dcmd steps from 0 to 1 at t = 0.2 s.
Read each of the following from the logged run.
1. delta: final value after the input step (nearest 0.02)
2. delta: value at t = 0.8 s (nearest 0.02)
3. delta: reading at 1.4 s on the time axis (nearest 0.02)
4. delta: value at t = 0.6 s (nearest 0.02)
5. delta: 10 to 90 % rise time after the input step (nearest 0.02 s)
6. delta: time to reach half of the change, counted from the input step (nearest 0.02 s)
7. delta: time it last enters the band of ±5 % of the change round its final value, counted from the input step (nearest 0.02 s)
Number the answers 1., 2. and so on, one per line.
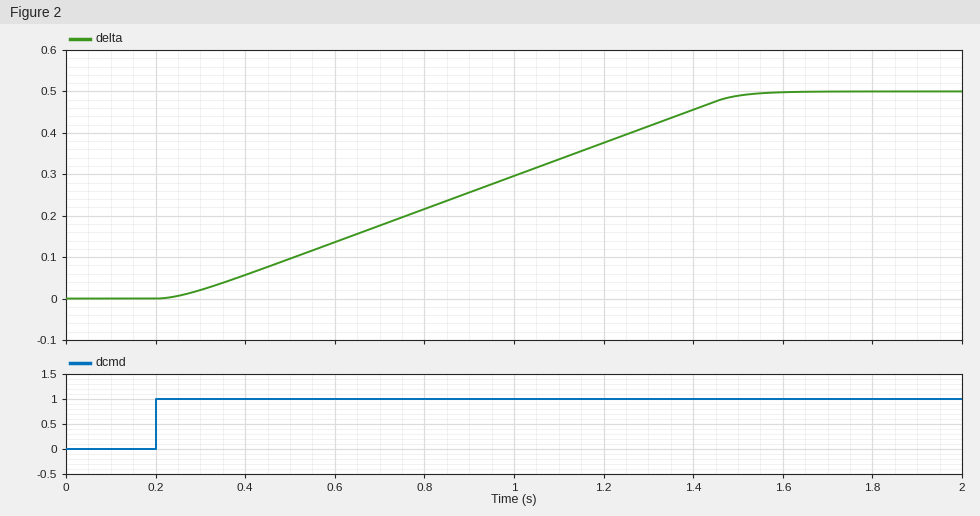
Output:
1. 0.50
2. 0.22
3. 0.46
4. 0.14
5. 1.00 s
6. 0.68 s
7. 1.24 s
